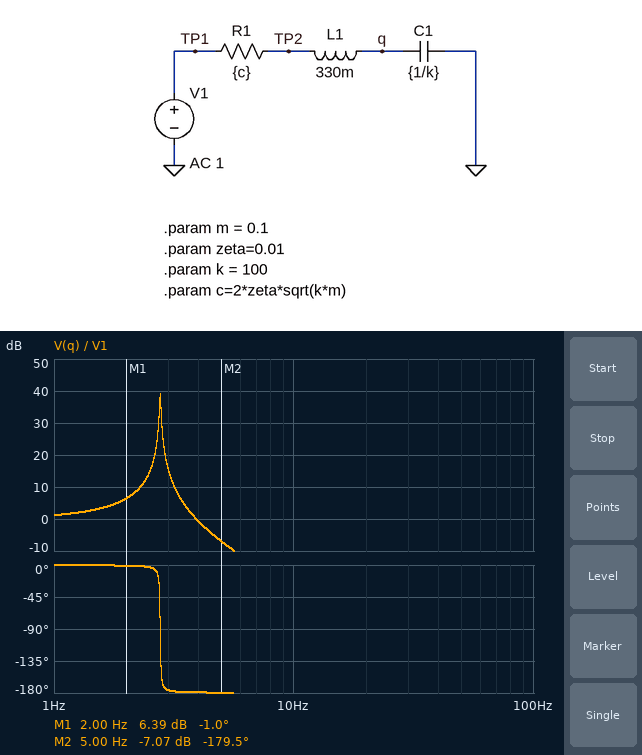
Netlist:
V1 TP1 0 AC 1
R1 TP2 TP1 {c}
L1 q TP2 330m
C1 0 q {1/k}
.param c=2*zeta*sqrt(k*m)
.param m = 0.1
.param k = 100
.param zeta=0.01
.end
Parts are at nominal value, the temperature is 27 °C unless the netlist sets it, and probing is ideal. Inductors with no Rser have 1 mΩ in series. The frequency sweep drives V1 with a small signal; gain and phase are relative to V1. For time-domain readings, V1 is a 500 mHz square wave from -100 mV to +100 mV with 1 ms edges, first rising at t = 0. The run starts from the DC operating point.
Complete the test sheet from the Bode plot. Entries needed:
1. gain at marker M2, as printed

-7.07 dB
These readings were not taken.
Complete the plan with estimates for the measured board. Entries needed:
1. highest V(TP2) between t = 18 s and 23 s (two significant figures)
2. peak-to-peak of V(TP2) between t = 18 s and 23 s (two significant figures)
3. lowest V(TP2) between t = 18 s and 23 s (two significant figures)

100 mV
200 mV
-100 mV
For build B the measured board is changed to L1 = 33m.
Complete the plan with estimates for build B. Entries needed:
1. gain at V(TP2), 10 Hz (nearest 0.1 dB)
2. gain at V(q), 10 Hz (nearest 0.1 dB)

-0.1 dB
10.3 dB
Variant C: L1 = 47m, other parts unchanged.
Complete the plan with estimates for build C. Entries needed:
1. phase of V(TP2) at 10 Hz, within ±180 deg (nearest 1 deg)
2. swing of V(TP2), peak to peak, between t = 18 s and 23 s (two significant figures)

3 deg
210 mV
